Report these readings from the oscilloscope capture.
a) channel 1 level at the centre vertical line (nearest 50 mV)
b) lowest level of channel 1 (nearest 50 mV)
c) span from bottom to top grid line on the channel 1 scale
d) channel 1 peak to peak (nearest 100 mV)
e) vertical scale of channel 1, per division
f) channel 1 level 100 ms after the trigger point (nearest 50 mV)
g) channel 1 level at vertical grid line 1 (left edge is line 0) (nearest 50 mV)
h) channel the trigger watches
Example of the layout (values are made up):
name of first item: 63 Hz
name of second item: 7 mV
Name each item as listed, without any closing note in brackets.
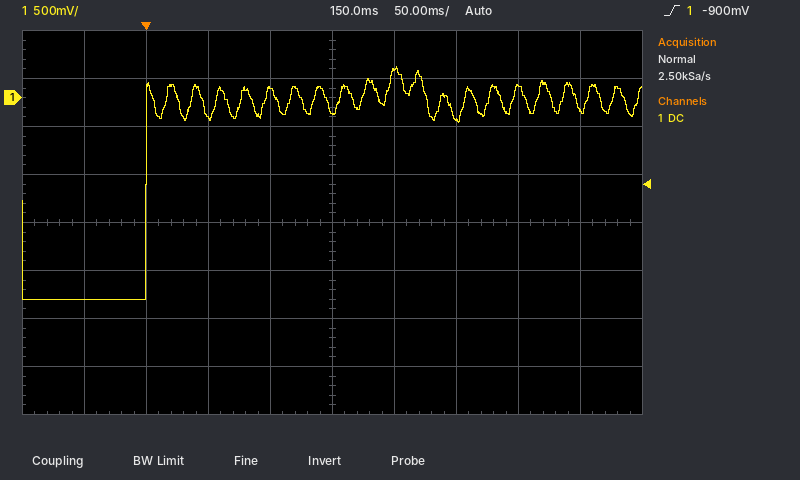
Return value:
channel 1 level at the centre vertical line: -150 mV
lowest level of channel 1: -2.10 V
span from bottom to top grid line on the channel 1 scale: 4 V
channel 1 peak to peak: 2.40 V
vertical scale of channel 1, per division: 500 mV
channel 1 level 100 ms after the trigger point: 100 mV
channel 1 level at vertical grid line 1 (left edge is line 0): -2.10 V
channel the trigger watches: channel 1
